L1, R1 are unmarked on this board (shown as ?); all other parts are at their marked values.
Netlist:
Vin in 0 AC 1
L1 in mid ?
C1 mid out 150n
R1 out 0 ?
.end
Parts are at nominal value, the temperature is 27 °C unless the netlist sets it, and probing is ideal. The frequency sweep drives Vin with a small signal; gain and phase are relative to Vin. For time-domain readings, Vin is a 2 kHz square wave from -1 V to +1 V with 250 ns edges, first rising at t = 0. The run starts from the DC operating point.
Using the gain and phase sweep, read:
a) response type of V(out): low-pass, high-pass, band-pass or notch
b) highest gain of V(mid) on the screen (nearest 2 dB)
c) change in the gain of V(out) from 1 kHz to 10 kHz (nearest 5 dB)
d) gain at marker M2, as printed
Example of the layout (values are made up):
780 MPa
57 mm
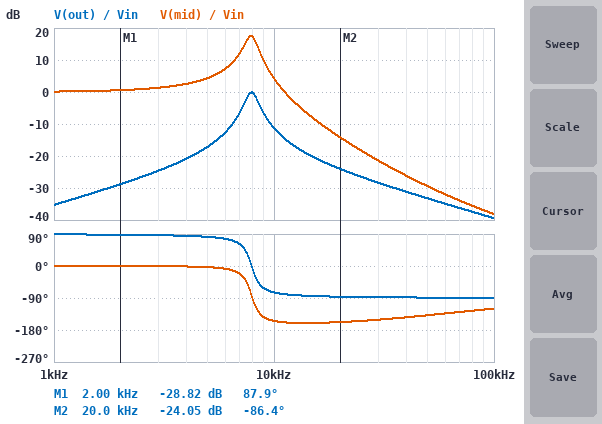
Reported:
band-pass
18 dB
25 dB
-24.05 dB
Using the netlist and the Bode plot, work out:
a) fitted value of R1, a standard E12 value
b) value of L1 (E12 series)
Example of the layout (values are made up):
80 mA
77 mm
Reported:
18 Ω
2.7 mH
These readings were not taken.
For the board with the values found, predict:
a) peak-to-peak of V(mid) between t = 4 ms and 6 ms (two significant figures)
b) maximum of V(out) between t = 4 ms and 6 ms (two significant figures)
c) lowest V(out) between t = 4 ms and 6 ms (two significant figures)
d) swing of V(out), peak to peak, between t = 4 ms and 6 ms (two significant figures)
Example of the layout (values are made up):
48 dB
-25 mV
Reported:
4.3 V
170 mV
-170 mV
340 mV
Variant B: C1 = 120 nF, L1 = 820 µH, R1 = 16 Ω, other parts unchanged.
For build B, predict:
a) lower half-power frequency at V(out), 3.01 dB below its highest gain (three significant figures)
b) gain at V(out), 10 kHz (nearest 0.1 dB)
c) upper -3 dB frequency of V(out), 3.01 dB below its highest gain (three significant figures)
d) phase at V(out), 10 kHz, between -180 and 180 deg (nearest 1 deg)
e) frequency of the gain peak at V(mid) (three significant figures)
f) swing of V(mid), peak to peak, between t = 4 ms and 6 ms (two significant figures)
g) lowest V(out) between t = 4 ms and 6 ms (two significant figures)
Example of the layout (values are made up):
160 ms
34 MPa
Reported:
14.6 kHz
-14.3 dB
17.7 kHz
79 deg
15.9 kHz
4.8 V
-310 mV
